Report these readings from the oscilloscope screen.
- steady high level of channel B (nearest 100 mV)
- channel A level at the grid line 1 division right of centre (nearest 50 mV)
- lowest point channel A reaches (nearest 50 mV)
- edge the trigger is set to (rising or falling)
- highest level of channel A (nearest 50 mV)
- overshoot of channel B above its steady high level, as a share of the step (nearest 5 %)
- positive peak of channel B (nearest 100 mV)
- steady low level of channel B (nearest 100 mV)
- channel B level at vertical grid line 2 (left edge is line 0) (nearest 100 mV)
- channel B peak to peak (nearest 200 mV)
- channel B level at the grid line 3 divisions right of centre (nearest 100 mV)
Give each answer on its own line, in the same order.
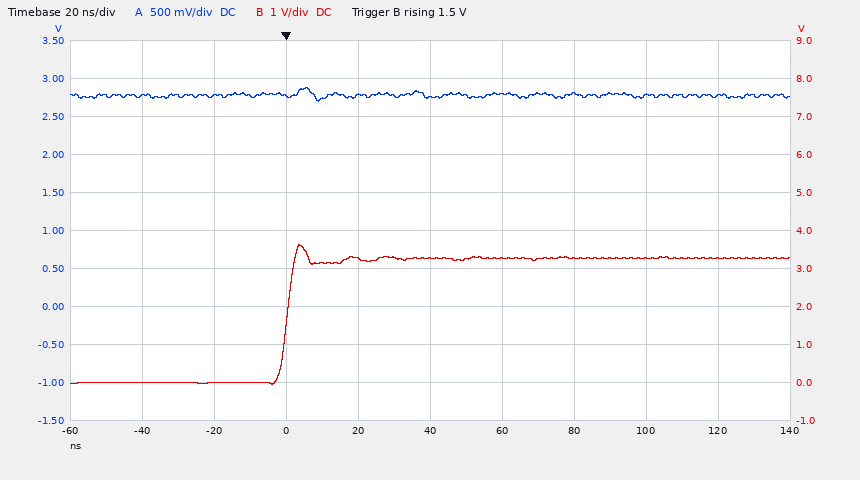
3.3 V
2.80 V
2.70 V
rising
2.90 V
10 %
3.6 V
0.0 V
0.0 V
3.6 V
3.3 V
